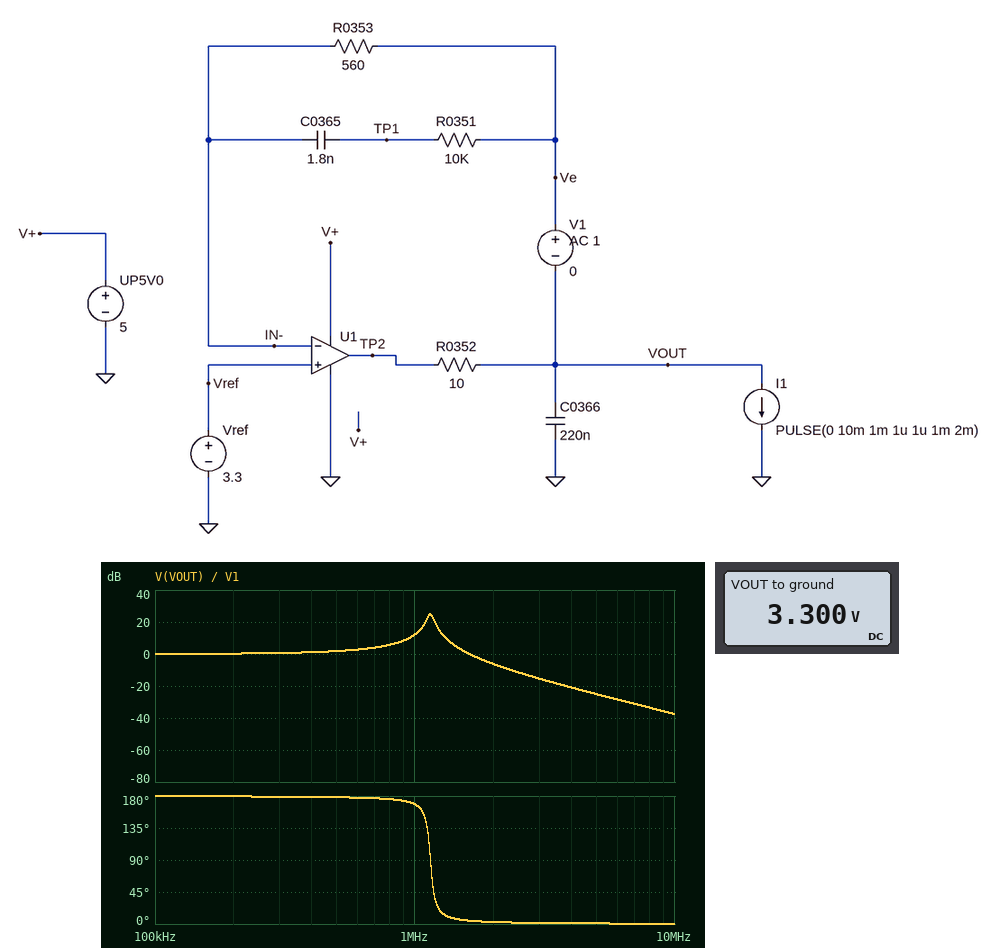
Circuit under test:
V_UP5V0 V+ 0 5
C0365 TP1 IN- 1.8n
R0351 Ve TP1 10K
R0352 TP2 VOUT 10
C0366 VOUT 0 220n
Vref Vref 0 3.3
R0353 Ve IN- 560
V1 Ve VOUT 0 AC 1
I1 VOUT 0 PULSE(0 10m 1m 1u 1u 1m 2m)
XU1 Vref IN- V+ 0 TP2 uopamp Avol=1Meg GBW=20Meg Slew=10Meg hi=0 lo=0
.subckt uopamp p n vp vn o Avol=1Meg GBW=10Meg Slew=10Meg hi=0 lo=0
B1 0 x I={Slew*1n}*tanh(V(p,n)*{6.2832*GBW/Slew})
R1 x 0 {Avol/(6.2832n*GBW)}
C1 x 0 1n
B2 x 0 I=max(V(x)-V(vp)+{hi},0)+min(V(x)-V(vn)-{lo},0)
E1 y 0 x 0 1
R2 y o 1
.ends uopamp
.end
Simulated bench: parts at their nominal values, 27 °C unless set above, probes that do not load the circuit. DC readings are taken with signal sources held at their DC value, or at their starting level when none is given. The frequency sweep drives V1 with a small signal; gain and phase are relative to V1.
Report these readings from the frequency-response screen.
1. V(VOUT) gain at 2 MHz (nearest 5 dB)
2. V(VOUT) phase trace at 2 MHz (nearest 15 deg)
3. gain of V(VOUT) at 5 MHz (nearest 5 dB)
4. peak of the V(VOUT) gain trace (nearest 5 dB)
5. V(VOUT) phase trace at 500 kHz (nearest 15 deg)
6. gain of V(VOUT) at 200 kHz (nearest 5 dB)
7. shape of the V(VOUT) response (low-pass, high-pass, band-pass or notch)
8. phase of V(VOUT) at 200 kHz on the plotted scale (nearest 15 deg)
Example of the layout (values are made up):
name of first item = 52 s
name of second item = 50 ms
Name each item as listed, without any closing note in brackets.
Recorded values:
V(VOUT) gain at 2 MHz = -5 dB
V(VOUT) phase trace at 2 MHz = 0 deg
gain of V(VOUT) at 5 MHz = -25 dB
peak of the V(VOUT) gain trace = 25 dB
V(VOUT) phase trace at 500 kHz = 180 deg
gain of V(VOUT) at 200 kHz = 0 dB
shape of the V(VOUT) response = low-pass
phase of V(VOUT) at 200 kHz on the plotted scale = 180 deg
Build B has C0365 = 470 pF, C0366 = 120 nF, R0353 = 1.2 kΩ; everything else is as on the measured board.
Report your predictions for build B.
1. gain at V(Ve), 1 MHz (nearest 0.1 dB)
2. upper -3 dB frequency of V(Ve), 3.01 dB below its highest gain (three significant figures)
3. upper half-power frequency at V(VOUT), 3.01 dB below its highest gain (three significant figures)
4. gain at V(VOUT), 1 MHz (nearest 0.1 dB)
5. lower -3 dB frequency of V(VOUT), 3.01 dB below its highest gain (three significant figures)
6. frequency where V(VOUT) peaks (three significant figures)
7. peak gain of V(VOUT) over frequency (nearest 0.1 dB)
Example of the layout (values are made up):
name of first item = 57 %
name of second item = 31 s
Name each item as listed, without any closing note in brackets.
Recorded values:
gain at V(Ve), 1 MHz = -3.0 dB
upper -3 dB frequency of V(Ve), 3.01 dB below its highest gain = 1.62 MHz
upper half-power frequency at V(VOUT), 3.01 dB below its highest gain = 1.61 MHz
gain at V(VOUT), 1 MHz = 4.6 dB
lower -3 dB frequency of V(VOUT), 3.01 dB below its highest gain = 1.49 MHz
frequency where V(VOUT) peaks = 1.55 MHz
peak gain of V(VOUT) over frequency = 22.2 dB
